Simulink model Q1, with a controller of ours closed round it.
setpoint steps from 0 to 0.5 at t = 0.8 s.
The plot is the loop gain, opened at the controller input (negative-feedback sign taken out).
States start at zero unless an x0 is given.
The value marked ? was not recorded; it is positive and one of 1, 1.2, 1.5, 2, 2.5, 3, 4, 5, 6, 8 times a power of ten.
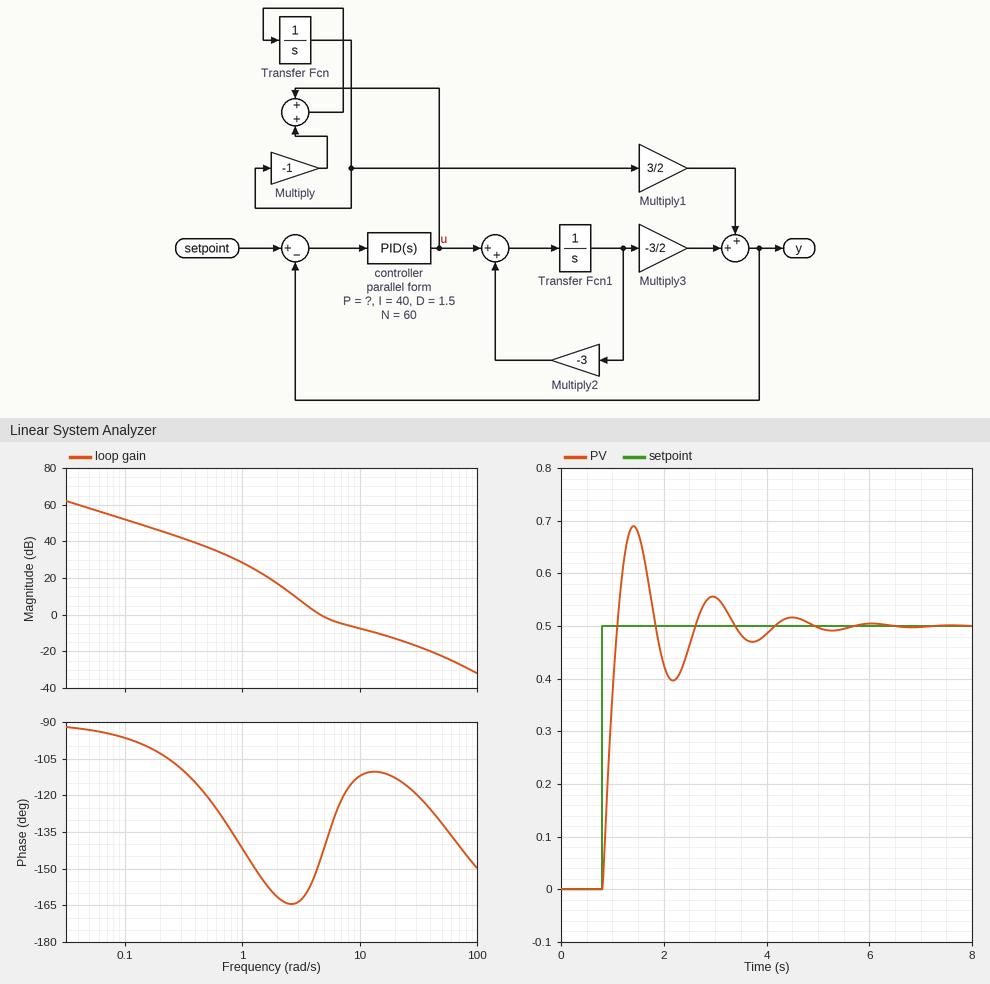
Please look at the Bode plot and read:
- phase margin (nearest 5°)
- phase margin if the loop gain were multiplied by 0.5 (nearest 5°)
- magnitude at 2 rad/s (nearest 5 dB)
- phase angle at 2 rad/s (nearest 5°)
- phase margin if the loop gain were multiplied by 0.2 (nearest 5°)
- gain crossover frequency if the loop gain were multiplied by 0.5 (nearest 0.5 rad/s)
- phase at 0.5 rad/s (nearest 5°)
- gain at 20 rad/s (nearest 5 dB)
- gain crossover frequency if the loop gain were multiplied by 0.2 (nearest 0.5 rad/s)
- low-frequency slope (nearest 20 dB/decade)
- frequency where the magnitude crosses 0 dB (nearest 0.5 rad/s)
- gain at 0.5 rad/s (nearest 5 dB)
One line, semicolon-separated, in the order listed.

35°; 20°; 15 dB; -160°; 15°; 3.5 rad/s; -120°; -15 dB; 2.5 rad/s; -20 dB/decade; 4.5 rad/s; 35 dB
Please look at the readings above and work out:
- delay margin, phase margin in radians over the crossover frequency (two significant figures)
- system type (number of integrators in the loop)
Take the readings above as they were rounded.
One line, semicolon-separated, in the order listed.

0.14 s; 1
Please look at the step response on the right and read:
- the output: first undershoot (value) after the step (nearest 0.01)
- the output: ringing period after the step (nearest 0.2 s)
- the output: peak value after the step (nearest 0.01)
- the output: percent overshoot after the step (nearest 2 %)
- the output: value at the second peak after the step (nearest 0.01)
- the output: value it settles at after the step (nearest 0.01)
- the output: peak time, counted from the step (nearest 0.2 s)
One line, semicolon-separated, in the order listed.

0.40; 1.6 s; 0.69; 38 %; 0.56; 0.50; 0.6 s
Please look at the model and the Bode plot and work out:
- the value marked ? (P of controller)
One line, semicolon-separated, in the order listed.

8
